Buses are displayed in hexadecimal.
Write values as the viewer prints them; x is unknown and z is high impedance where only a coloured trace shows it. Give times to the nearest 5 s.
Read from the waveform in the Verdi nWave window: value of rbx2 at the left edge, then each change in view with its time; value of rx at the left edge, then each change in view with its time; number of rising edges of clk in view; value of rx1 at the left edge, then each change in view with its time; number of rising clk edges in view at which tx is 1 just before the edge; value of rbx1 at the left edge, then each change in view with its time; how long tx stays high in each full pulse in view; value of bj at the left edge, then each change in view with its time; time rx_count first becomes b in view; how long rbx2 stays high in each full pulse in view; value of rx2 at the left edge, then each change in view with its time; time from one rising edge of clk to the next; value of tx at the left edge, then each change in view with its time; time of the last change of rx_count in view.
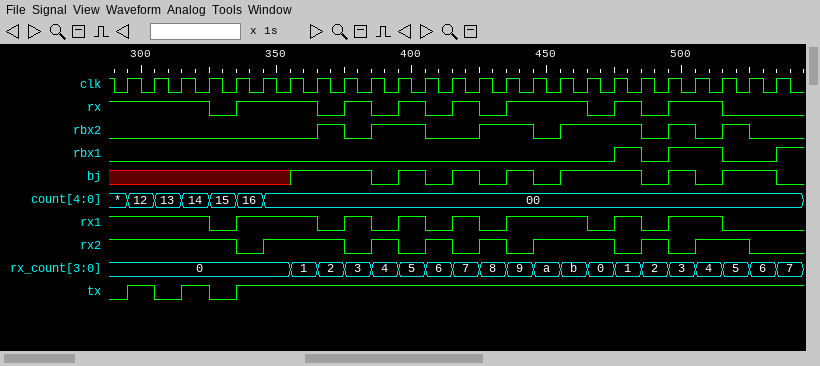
0, 1 at 365 s, 0 at 375 s, 1 at 385 s, 0 at 405 s, 1 at 425 s, 0 at 445 s, 1 at 455 s, 0 at 485 s, 1 at 495 s, 0 at 505 s, 1 at 515 s, 0 at 525 s
1, 0 at 325 s, 1 at 335 s, 0 at 365 s, 1 at 375 s, 0 at 385 s, 1 at 395 s, 0 at 405 s, 1 at 415 s, 0 at 425 s, 1 at 435 s, 0 at 465 s, 1 at 475 s, 0 at 485 s, 1 at 495 s, 0 at 515 s
25
1, 0 at 325 s, 1 at 335 s, 0 at 365 s, 1 at 375 s, 0 at 385 s, 1 at 395 s, 0 at 405 s, 1 at 415 s, 0 at 425 s, 1 at 435 s, 0 at 465 s, 1 at 475 s, 0 at 485 s, 1 at 495 s, 0 at 515 s
22
0, 1 at 475 s, 0 at 485 s, 1 at 495 s, 0 at 515 s, 1 at 535 s
10 s, 10 s
x, 1 at 355 s, 0 at 385 s, 1 at 395 s, 0 at 405 s, 1 at 415 s, 0 at 425 s, 1 at 435 s, 0 at 445 s, 1 at 455 s, 0 at 485 s, 1 at 495 s, 0 at 505 s, 1 at 515 s, 0 at 535 s
455 s
10 s, 20 s, 20 s, 30 s, 10 s, 10 s
1, 0 at 335 s, 1 at 345 s, 0 at 375 s, 1 at 385 s, 0 at 395 s, 1 at 405 s, 0 at 415 s, 1 at 425 s, 0 at 435 s, 1 at 445 s, 0 at 475 s, 1 at 485 s, 0 at 495 s, 1 at 505 s, 0 at 525 s
10 s
0, 1 at 295 s, 0 at 305 s, 1 at 315 s, 0 at 325 s, 1 at 335 s
535 s
